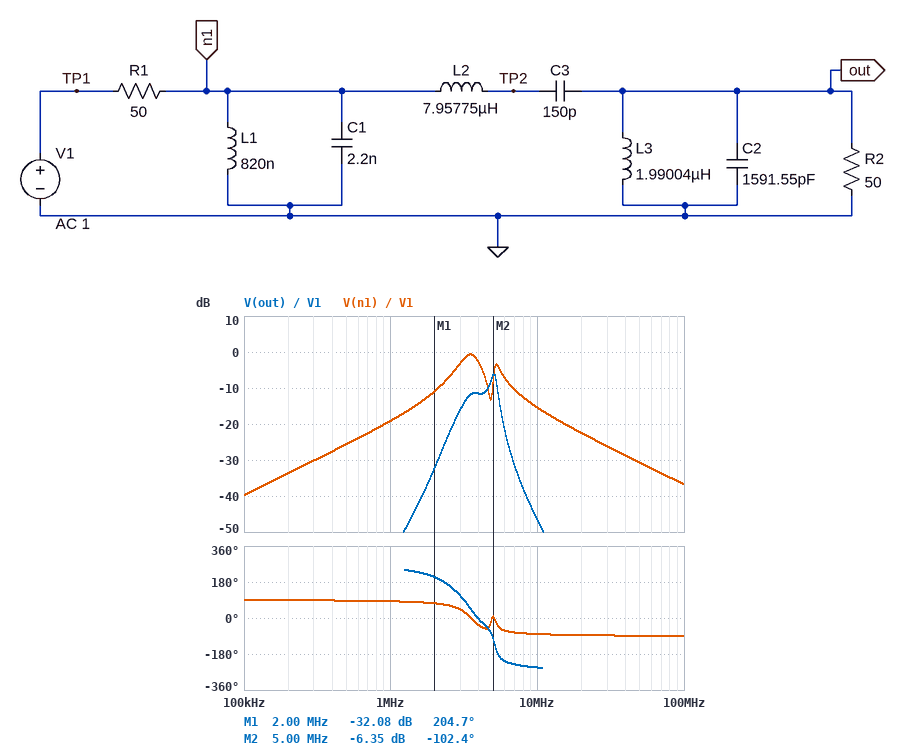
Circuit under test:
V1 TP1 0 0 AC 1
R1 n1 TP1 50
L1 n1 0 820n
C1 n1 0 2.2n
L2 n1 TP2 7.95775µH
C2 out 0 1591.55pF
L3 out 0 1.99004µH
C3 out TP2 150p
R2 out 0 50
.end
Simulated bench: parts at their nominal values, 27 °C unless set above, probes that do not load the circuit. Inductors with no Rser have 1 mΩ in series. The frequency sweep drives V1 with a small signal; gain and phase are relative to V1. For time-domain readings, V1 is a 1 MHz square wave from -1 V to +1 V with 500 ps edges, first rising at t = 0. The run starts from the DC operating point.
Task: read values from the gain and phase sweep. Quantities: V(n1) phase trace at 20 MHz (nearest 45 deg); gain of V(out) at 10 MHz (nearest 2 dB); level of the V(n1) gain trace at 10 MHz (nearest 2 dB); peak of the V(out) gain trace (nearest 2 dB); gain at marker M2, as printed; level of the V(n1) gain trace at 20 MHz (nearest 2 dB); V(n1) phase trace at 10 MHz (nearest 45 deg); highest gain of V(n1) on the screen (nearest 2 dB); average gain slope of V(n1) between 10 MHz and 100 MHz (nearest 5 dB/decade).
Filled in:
-90 deg
-46 dB
-16 dB
-6 dB
-6.35 dB
-22 dB
-90 deg
0 dB
-20 dB/decade
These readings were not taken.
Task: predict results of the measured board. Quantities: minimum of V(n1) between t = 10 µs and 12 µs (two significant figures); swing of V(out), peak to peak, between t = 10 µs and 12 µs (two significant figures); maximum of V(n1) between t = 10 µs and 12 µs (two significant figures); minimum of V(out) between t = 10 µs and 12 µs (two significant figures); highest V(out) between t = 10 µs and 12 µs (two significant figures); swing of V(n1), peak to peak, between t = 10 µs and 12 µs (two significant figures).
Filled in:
-620 mV
380 mV
620 mV
-190 mV
190 mV
1.2 V
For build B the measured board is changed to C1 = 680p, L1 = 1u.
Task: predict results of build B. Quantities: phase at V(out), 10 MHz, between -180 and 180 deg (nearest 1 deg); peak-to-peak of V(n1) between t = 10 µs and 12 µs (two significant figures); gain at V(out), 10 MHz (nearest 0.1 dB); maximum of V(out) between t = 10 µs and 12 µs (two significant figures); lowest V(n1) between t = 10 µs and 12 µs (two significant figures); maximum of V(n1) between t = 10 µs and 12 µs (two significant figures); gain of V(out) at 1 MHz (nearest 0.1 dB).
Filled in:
142 deg
1.7 V
-35.1 dB
130 mV
-850 mV
850 mV
-55.0 dB
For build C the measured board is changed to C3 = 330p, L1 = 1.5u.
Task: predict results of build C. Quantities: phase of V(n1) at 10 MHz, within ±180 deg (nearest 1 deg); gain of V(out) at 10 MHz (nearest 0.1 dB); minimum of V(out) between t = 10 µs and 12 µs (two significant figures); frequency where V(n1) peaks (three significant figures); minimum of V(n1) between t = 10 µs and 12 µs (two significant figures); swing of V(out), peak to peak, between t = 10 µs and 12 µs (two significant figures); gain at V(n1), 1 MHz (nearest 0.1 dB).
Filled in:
-81 deg
-48.4 dB
-220 mV
2.20 MHz
-590 mV
450 mV
-13.3 dB
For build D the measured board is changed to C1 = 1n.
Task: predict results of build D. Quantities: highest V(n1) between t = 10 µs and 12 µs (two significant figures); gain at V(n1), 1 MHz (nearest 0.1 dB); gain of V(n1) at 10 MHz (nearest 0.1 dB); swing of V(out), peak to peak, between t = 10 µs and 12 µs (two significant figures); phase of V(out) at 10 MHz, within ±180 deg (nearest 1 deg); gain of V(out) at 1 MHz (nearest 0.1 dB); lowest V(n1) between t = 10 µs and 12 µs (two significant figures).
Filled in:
670 mV
-19.5 dB
-7.1 dB
270 mV
129 deg
-56.7 dB
-670 mV
